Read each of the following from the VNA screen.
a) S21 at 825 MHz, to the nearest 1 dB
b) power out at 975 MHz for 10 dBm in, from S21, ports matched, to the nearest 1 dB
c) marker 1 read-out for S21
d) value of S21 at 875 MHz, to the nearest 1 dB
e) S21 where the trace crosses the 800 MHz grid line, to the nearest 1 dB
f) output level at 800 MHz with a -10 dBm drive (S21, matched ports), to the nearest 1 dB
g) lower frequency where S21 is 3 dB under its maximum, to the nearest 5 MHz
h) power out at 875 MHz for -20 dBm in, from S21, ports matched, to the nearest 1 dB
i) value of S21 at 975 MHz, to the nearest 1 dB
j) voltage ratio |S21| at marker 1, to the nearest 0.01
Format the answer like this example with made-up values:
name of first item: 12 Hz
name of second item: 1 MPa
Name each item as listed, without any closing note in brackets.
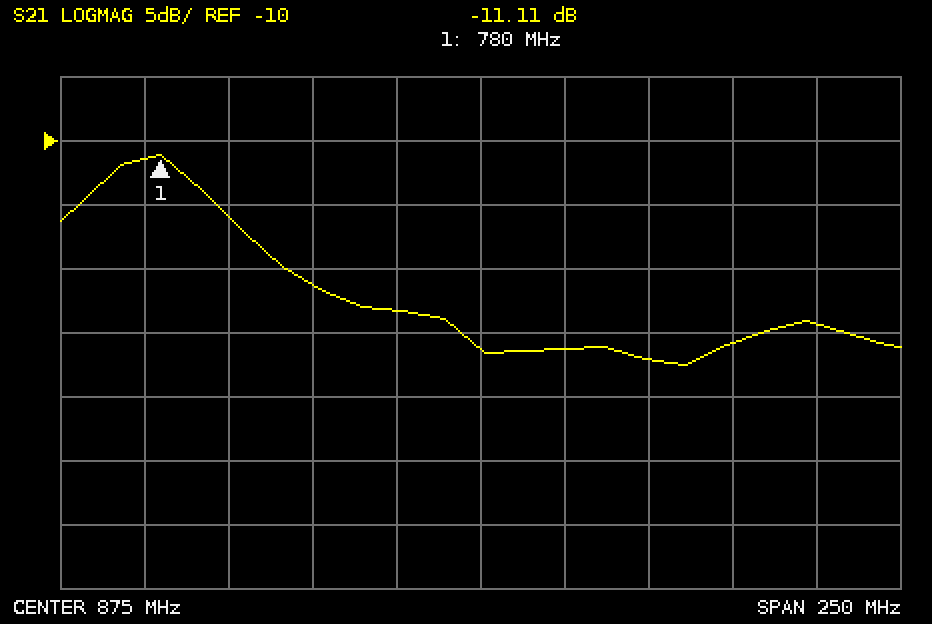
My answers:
S21 at 825 MHz, to the nearest 1 dB: -21 dB
power out at 975 MHz for 10 dBm in, from S21, ports matched, to the nearest 1 dB: -14 dBm
marker 1 read-out for S21: -11.11 dB
value of S21 at 875 MHz, to the nearest 1 dB: -26 dB
S21 where the trace crosses the 800 MHz grid line, to the nearest 1 dB: -16 dB
output level at 800 MHz with a -10 dBm drive (S21, matched ports), to the nearest 1 dB: -26 dBm
lower frequency where S21 is 3 dB under its maximum, to the nearest 5 MHz: 760 MHz
power out at 875 MHz for -20 dBm in, from S21, ports matched, to the nearest 1 dB: -46 dBm
value of S21 at 975 MHz, to the nearest 1 dB: -24 dB
voltage ratio |S21| at marker 1, to the nearest 0.01: 0.28
